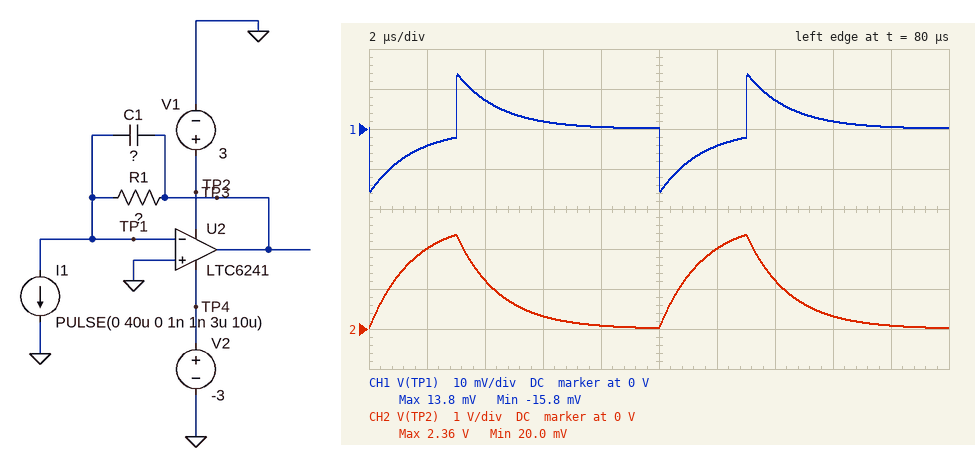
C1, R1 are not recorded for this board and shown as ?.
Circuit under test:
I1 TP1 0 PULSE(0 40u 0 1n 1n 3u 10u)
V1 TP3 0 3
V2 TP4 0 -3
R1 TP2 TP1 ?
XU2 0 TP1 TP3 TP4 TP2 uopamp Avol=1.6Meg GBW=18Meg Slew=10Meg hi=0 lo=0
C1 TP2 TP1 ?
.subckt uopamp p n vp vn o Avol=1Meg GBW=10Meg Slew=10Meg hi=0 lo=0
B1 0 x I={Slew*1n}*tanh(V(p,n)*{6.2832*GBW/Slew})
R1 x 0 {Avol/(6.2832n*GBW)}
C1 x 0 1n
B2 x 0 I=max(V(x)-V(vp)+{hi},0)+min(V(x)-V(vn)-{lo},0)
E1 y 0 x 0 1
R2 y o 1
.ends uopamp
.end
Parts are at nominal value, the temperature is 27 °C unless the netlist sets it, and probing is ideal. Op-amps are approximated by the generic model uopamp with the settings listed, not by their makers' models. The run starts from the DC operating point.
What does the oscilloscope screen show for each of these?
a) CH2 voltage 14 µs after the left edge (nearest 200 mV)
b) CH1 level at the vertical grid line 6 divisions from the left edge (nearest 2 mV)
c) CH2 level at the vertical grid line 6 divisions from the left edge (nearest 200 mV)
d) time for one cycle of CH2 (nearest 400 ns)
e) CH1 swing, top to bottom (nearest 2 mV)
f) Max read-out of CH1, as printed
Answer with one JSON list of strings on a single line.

["1.2 V", "-4 mV", "2.0 V", "10.0 µs", "30 mV", "13.8 mV"]
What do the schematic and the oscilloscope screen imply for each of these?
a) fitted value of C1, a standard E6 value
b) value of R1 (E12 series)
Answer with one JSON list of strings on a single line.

["22 pF", "68 kΩ"]
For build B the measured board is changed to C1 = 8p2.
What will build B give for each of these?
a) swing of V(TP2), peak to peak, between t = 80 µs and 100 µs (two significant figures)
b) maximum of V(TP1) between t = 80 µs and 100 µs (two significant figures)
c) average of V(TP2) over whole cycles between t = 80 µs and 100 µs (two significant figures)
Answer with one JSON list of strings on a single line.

["2.7 V", "44 mV", "820 mV"]
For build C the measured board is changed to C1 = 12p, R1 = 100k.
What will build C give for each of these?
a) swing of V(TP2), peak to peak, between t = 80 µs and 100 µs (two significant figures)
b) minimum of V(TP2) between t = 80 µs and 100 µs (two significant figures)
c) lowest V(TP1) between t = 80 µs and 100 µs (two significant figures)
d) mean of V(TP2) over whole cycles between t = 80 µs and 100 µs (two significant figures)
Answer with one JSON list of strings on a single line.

["3.0 V", "11 mV", "-660 mV", "1.1 V"]
